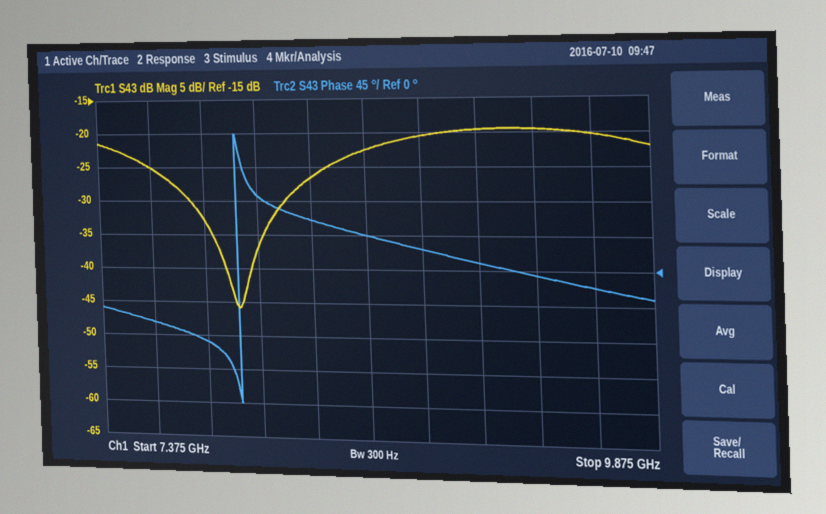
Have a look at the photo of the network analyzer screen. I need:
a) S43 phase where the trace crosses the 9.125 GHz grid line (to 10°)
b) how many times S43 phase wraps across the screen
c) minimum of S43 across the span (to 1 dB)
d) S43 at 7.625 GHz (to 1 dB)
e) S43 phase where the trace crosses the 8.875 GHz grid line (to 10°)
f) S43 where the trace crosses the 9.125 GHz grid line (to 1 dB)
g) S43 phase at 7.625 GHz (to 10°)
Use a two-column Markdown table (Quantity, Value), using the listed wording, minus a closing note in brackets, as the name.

| Quantity | Value |
|---|---|
| S43 phase where the trace crosses the 9.125 GHz grid line | 10° |
| how many times S43 phase wraps across the screen | 1 |
| minimum of S43 across the span | -46 dB |
| S43 at 7.625 GHz | -25 dB |
| S43 phase where the trace crosses the 8.875 GHz grid line | 30° |
| S43 where the trace crosses the 9.125 GHz grid line | -20 dB |
| S43 phase at 7.625 GHz | -70° |
